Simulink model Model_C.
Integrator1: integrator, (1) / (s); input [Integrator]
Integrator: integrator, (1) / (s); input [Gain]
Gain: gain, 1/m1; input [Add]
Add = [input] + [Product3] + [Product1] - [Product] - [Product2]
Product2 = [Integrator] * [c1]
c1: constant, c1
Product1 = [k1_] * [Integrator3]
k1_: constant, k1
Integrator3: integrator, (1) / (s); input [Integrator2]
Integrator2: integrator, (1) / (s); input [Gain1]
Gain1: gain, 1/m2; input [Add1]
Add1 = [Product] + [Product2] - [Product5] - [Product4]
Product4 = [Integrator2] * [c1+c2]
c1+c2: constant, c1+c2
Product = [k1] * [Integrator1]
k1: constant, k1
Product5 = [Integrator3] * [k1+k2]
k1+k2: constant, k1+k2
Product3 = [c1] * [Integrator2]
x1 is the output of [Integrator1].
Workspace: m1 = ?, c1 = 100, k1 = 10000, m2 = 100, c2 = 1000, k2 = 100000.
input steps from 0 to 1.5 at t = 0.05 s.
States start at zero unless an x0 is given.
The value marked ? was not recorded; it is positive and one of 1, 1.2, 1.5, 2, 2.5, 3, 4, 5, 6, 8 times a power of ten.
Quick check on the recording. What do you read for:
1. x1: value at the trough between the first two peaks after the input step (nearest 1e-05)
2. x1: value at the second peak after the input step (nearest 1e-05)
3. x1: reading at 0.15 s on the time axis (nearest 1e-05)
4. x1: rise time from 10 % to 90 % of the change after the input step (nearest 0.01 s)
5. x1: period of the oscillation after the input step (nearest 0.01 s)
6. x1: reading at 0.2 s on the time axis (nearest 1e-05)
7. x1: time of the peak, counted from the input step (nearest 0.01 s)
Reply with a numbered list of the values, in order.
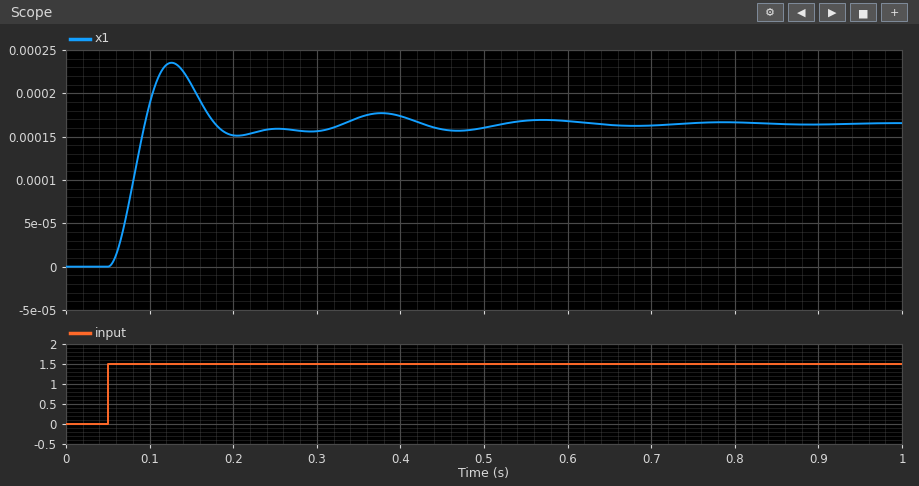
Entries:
1. 0.00015
2. 0.00018
3. 0.00021
4. 0.03 s
5. 0.25 s
6. 0.00015
7. 0.08 s
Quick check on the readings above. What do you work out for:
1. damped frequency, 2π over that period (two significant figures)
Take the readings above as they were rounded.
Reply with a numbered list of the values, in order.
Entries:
1. 25 rad/s
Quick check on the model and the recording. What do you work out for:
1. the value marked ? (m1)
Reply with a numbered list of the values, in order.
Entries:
1. 5
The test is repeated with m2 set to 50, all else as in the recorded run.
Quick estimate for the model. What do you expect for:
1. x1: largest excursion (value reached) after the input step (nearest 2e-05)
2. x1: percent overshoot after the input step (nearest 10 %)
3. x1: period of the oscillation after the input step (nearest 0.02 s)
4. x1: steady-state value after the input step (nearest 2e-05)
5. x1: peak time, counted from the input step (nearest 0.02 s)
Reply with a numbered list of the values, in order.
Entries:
1. 0.00024
2. 50 %
3. 0.18 s
4. 0.00016
5. 0.08 s
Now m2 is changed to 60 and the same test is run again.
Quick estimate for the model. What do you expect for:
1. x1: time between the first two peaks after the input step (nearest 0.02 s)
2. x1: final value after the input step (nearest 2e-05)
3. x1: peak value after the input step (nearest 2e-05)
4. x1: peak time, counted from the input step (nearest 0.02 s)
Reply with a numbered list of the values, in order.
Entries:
1. 0.18 s
2. 0.00016
3. 0.00024
4. 0.08 s
